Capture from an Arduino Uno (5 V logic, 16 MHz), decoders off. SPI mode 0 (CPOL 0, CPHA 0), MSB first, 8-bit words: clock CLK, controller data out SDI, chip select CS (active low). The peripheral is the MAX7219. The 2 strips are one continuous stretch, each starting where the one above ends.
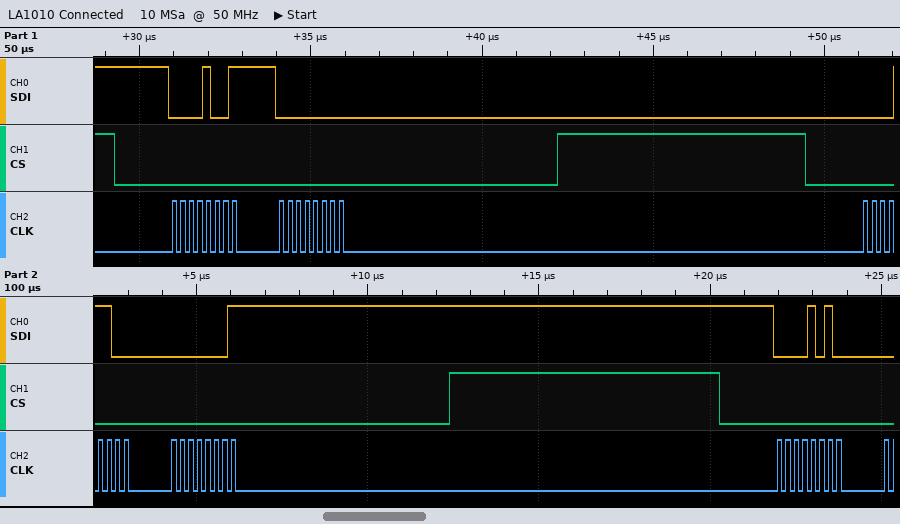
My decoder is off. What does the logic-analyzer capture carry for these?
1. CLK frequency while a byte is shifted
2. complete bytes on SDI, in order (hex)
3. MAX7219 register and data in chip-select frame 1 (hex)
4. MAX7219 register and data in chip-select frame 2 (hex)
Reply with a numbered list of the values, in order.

1. 4 MHz
2. 0x09 0x00 0x0C 0x01 0x0A
3. register 0x9, data 0x00
4. register 0xC, data 0x01
